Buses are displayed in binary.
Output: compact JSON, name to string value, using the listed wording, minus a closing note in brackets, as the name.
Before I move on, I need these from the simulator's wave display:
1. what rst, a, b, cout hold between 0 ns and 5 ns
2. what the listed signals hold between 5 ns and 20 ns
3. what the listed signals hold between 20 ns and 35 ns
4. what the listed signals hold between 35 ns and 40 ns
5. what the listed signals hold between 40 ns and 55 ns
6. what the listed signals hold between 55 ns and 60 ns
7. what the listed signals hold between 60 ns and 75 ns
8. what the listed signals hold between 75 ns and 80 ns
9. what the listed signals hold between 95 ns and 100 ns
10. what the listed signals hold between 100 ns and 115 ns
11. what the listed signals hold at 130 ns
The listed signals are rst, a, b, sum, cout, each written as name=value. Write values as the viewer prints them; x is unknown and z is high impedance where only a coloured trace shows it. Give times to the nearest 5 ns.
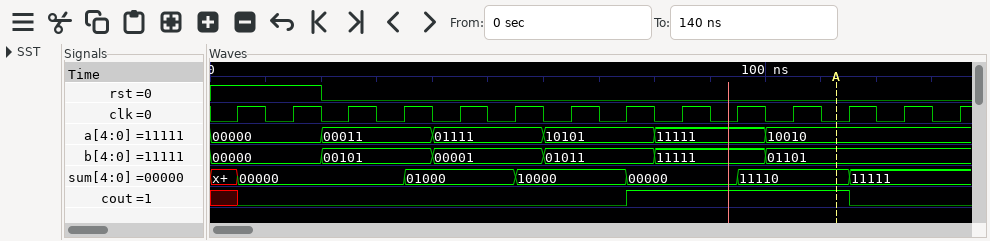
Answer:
{"what rst, a, b, cout hold between 0 ns and 5 ns": "rst=1, a=00000, b=00000, cout=x", "what the listed signals hold between 5 ns and 20 ns": "rst=1, a=00000, b=00000, sum=00000, cout=0", "what the listed signals hold between 20 ns and 35 ns": "rst=0, a=00011, b=00101, sum=00000, cout=0", "what the listed signals hold between 35 ns and 40 ns": "rst=0, a=00011, b=00101, sum=01000, cout=0", "what the listed signals hold between 40 ns and 55 ns": "rst=0, a=01111, b=00001, sum=01000, cout=0", "what the listed signals hold between 55 ns and 60 ns": "rst=0, a=01111, b=00001, sum=10000, cout=0", "what the listed signals hold between 60 ns and 75 ns": "rst=0, a=10101, b=01011, sum=10000, cout=0", "what the listed signals hold between 75 ns and 80 ns": "rst=0, a=10101, b=01011, sum=00000, cout=1", "what the listed signals hold between 95 ns and 100 ns": "rst=0, a=11111, b=11111, sum=11110, cout=1", "what the listed signals hold between 100 ns and 115 ns": "rst=0, a=10010, b=01101, sum=11110, cout=1", "what the listed signals hold at 130 ns": "rst=0, a=10010, b=01101, sum=11111, cout=0"}
